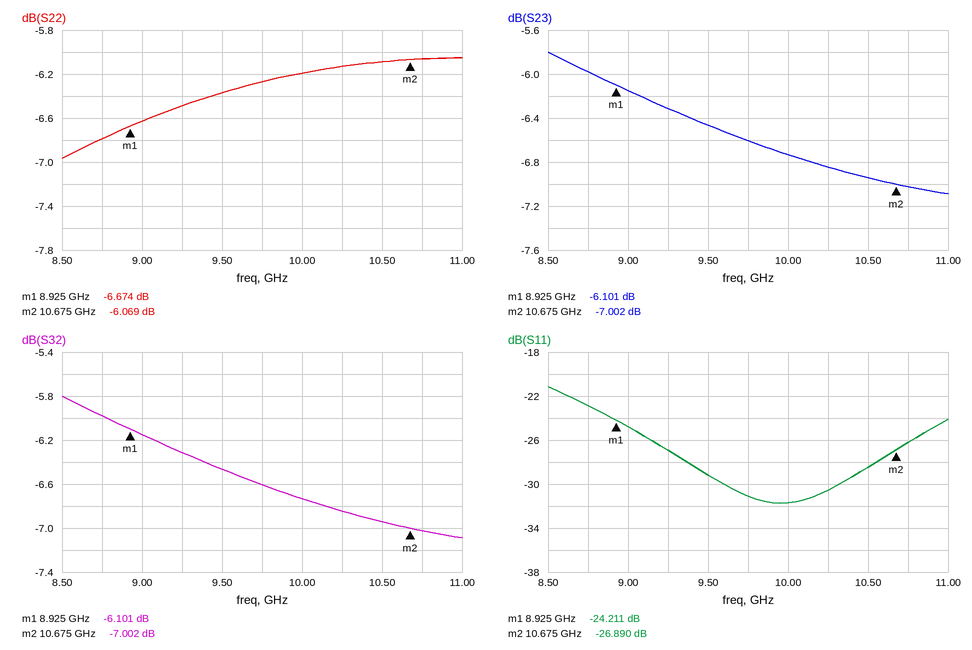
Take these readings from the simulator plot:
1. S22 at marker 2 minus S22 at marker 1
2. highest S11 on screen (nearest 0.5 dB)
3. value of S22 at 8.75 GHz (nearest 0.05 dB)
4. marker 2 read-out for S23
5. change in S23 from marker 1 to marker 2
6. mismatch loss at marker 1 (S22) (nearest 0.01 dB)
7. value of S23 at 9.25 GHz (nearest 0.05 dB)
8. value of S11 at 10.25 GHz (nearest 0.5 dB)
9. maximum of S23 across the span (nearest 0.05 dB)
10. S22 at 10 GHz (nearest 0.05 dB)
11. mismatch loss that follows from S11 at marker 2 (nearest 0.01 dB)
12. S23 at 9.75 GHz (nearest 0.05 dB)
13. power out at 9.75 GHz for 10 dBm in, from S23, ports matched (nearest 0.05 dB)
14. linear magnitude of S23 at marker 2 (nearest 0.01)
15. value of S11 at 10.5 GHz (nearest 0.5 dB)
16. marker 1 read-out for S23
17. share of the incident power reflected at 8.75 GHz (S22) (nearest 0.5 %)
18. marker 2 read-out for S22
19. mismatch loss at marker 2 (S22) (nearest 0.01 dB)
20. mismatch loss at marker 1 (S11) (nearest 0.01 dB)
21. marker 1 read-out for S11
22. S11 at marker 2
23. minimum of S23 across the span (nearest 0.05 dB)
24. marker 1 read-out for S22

0.605 dB
-21.0 dB
-6.80 dB
-7.002 dB
-0.901 dB
1.05 dB
-6.30 dB
-30.5 dB
-5.80 dB
-6.20 dB
0.01 dB
-6.60 dB
3.40 dBm
0.45
-28.5 dB
-6.101 dB
21.0 %
-6.069 dB
1.23 dB
0.02 dB
-24.211 dB
-26.890 dB
-7.10 dB
-6.674 dB
